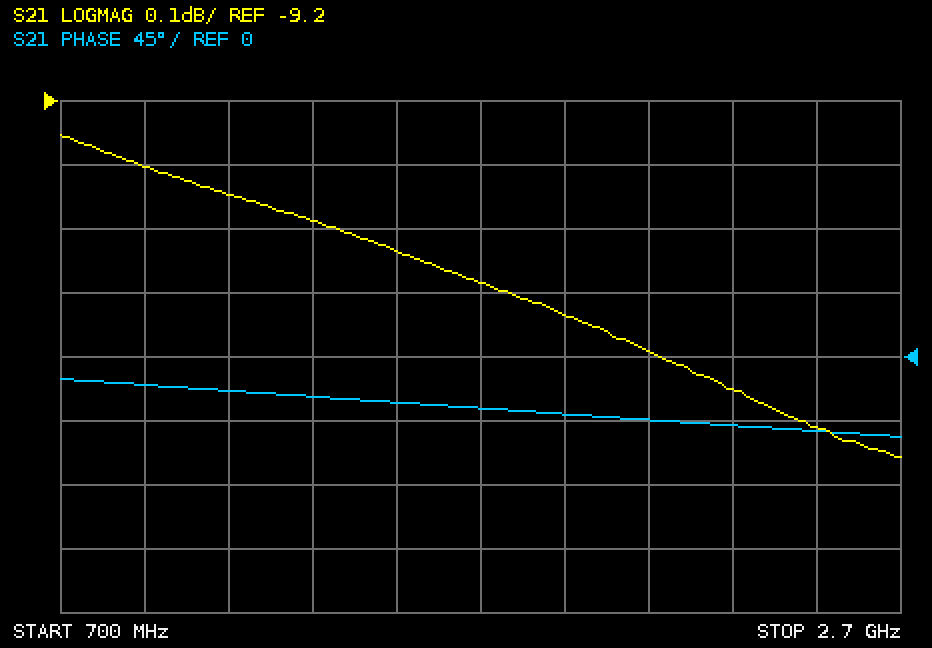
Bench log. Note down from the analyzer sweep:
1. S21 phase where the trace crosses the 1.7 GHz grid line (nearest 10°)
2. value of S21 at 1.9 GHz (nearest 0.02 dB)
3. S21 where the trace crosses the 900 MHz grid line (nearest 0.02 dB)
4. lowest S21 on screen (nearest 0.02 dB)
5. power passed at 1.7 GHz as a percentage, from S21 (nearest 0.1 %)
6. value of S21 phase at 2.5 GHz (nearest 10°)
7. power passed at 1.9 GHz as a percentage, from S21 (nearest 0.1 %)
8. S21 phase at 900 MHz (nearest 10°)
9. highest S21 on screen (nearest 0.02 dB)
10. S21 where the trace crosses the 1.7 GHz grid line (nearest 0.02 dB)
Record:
-40°
-9.54 dB
-9.30 dB
-9.76 dB
11.3 %
-50°
11.1 %
-20°
-9.26 dB
-9.48 dB
